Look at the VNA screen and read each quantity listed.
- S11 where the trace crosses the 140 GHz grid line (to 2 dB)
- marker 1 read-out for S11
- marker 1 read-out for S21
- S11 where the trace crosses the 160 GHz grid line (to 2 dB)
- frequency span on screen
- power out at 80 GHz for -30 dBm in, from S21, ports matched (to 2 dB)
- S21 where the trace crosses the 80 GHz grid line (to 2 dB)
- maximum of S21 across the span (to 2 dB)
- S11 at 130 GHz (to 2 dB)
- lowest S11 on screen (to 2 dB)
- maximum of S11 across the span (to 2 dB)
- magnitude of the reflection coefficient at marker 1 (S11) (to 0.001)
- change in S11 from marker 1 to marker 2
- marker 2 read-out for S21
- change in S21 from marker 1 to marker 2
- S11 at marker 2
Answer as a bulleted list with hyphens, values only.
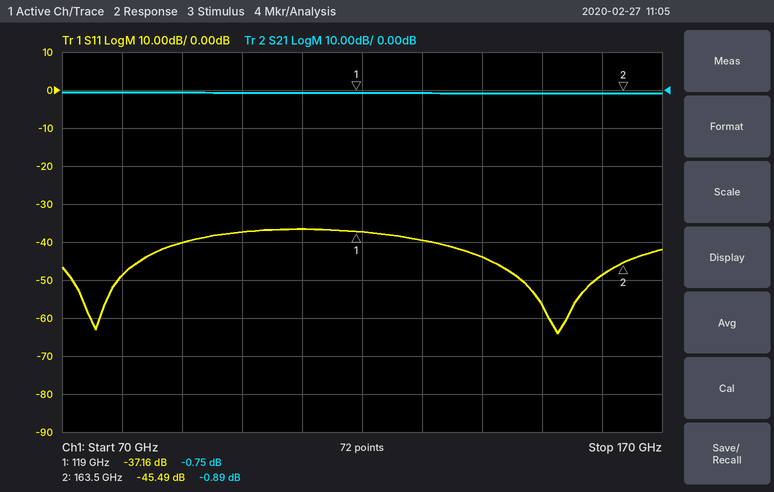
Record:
- -44 dB
- -37.16 dB
- -0.75 dB
- -48 dB
- 100 GHz
- -30 dBm
- 0 dB
- 0 dB
- -40 dB
- -64 dB
- -36 dB
- 0.014
- -8.33 dB
- -0.89 dB
- -0.14 dB
- -45.49 dB
